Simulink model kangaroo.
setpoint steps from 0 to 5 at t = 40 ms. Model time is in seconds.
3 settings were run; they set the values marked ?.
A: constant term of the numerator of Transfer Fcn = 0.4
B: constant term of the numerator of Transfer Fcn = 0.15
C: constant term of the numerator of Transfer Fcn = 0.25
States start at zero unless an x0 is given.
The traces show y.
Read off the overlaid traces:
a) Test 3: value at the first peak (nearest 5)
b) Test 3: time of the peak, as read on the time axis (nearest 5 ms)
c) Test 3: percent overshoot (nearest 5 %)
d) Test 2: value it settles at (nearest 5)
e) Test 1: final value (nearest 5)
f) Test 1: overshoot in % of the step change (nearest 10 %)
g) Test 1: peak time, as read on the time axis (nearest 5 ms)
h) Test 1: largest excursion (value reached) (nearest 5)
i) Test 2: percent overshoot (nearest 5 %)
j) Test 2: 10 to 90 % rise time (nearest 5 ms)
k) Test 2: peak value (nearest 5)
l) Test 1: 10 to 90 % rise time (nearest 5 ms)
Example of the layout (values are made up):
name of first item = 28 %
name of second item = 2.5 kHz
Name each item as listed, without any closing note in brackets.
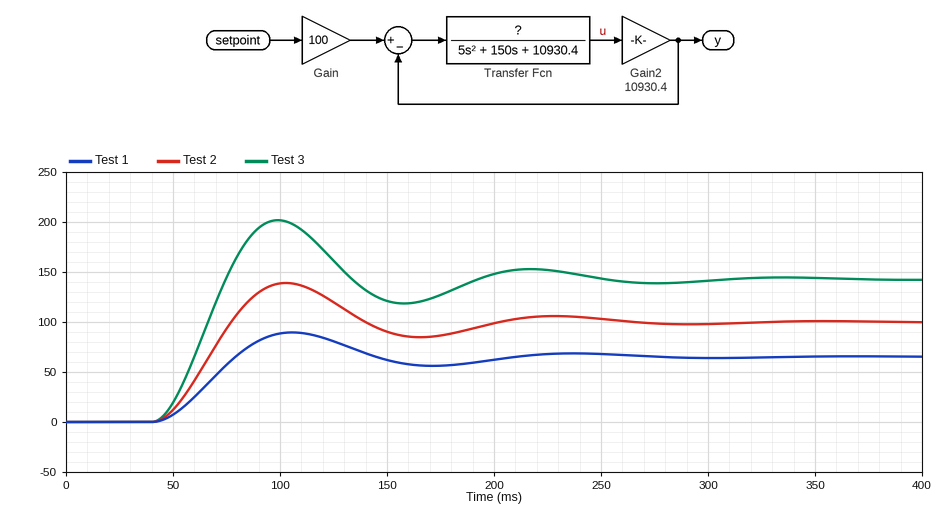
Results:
Test 3: value at the first peak = 200
Test 3: time of the peak, as read on the time axis = 100 ms
Test 3: percent overshoot = 40 %
Test 2: value it settles at = 100
Test 1: final value = 65
Test 1: overshoot in % of the step change = 40 %
Test 1: peak time, as read on the time axis = 105 ms
Test 1: largest excursion (value reached) = 90
Test 2: percent overshoot = 40 %
Test 2: 10 to 90 % rise time = 25 ms
Test 2: peak value = 140
Test 1: 10 to 90 % rise time = 25 ms
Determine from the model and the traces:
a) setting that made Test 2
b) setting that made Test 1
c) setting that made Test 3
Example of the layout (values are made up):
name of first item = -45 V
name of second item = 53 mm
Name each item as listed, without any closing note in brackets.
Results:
setting that made Test 2 = C
setting that made Test 1 = B
setting that made Test 3 = A
